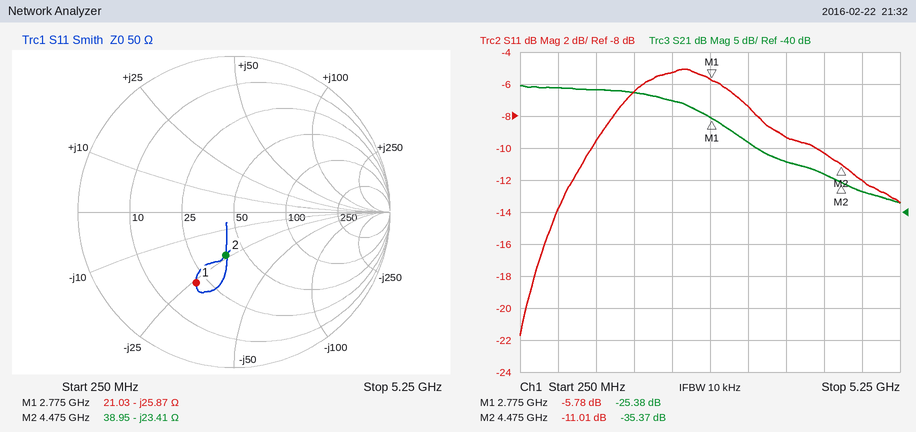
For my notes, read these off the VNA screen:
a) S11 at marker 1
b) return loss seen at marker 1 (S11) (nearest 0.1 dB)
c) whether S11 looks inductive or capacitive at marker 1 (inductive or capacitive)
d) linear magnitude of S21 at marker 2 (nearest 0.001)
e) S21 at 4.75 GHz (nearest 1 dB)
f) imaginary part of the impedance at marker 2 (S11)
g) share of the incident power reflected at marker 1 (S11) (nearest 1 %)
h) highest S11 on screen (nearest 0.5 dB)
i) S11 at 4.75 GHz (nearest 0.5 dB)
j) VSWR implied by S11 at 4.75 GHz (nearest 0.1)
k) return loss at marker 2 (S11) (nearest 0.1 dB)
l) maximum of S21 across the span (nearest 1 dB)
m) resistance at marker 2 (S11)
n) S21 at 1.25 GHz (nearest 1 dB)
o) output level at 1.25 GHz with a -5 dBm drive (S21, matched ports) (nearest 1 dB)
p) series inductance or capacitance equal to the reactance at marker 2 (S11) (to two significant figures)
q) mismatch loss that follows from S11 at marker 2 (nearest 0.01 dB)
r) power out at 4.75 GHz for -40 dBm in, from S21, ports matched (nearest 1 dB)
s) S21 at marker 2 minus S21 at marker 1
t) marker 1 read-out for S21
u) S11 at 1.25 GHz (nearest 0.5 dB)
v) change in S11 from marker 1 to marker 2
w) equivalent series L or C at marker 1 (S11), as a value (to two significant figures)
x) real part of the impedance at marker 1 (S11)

-5.78 dB
5.8 dB
capacitive
0.017
-37 dB
-23.41 Ω
26 %
-5.0 dB
-12.0 dB
1.7
11.0 dB
-20 dB
38.95 Ω
-21 dB
-26 dBm
1.5 pF
0.36 dB
-77 dBm
-9.99 dB
-25.38 dB
-9.5 dB
-5.23 dB
2.2 pF
21.03 Ω
